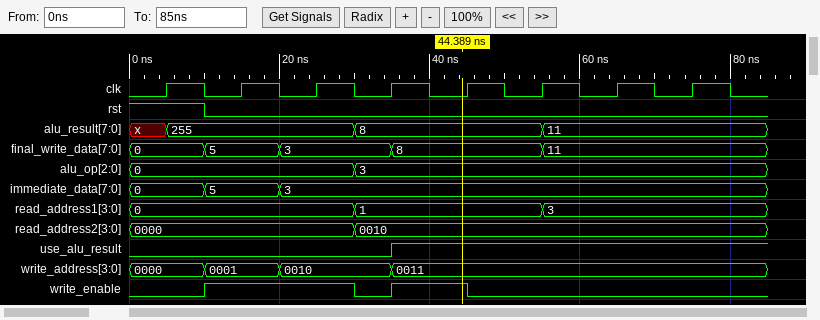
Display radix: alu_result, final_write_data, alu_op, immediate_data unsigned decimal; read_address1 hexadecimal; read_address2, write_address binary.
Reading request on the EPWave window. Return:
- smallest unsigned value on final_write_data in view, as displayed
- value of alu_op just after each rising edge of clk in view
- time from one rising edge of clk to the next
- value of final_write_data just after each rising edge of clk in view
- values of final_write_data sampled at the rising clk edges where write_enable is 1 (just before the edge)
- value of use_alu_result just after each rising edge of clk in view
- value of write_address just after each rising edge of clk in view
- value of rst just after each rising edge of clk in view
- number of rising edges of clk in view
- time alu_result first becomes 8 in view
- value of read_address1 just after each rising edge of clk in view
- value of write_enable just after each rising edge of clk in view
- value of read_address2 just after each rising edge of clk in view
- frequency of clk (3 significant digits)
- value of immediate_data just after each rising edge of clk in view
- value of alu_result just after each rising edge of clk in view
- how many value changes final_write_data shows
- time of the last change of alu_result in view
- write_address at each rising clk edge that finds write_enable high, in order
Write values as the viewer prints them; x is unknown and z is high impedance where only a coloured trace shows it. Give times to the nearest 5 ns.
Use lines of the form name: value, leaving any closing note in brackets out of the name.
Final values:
smallest unsigned value on final_write_data in view, as displayed: 0
value of alu_op just after each rising edge of clk in view: 0, 0, 0, 3, 3, 3, 3, 3
time from one rising edge of clk to the next: 10 ns
value of final_write_data just after each rising edge of clk in view: 0, 5, 3, 8, 8, 11, 11, 11
values of final_write_data sampled at the rising clk edges where write_enable is 1: 5, 3, 8
value of use_alu_result just after each rising edge of clk in view: 0 0 0 1 1 1 1 1
value of write_address just after each rising edge of clk in view: 0000, 0001, 0010, 0011, 0011, 0011, 0011, 0011
value of rst just after each rising edge of clk in view: 1 0 0 0 0 0 0 0
number of rising edges of clk in view: 8
time alu_result first becomes 8 in view: 30 ns
value of read_address1 just after each rising edge of clk in view: 0, 0, 0, 1, 1, 3, 3, 3
value of write_enable just after each rising edge of clk in view: 0 1 1 1 0 0 0 0
value of read_address2 just after each rising edge of clk in view: 0000, 0000, 0000, 0010, 0010, 0010, 0010, 0010
frequency of clk: 100 MHz
value of immediate_data just after each rising edge of clk in view: 0, 5, 3, 3, 3, 3, 3, 3
value of alu_result just after each rising edge of clk in view: 255, 255, 255, 8, 8, 11, 11, 11
how many value changes final_write_data shows: 4
time of the last change of alu_result in view: 55 ns
write_address at each rising clk edge that finds write_enable high, in order: 0001, 0010, 0011
